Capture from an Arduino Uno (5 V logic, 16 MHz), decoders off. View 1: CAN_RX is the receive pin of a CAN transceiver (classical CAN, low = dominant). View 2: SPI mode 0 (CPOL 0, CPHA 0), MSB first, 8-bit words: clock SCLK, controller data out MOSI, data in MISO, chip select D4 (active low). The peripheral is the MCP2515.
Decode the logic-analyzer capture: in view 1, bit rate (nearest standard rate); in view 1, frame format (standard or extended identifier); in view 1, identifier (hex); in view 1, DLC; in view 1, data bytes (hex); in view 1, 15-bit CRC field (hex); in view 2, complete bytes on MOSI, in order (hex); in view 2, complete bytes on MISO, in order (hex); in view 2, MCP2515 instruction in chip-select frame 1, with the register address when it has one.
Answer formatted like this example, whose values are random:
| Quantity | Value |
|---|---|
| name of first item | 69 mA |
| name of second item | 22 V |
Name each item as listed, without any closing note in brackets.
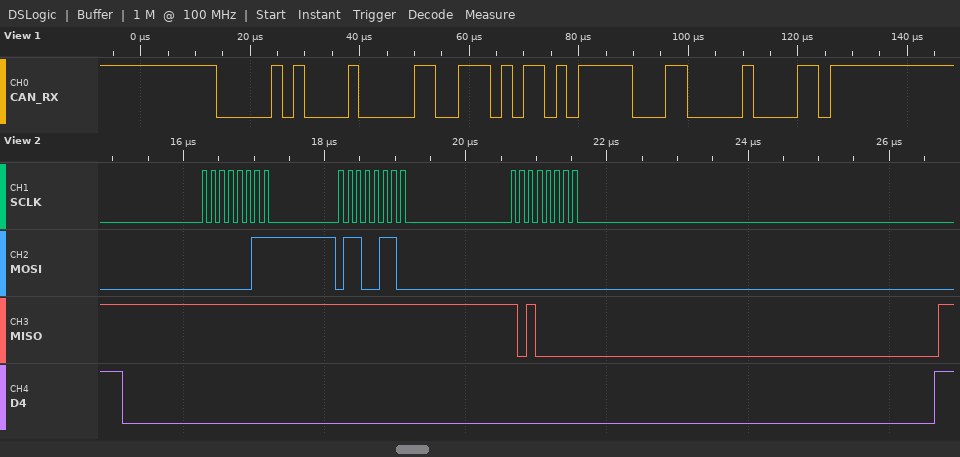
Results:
| Quantity | Value |
|---|---|
| in view 1, bit rate | 500 kbit/s |
| in view 1, frame format | standard |
| in view 1, identifier | 0x021 |
| in view 1, DLC | 2 |
| in view 1, data bytes | 75 AF |
| in view 1, 15-bit CRC field | 0x4C01 |
| in view 2, complete bytes on MOSI, in order | 03 66 00 |
| in view 2, complete bytes on MISO, in order | FF FF A0 |
| in view 2, MCP2515 instruction in chip-select frame 1, with the register address when it has one | READ 0x66 |
